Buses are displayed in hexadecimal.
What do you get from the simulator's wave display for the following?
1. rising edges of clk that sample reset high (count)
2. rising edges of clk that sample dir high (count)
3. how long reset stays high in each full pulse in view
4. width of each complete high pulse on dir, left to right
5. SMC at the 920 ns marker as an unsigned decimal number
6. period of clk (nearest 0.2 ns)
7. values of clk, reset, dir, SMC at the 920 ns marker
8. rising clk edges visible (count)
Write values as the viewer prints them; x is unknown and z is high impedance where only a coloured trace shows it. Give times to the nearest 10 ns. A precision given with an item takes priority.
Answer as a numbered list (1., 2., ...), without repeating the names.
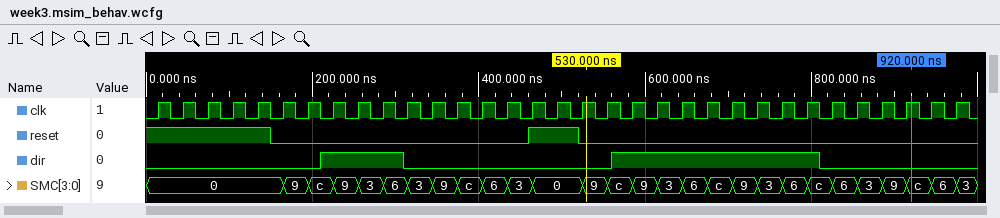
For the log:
1. 7
2. 11
3. 60 ns
4. 100 ns, 250 ns
5. 12
6. 30 ns
7. clk=1, reset=0, dir=0, SMC=c
8. 33
